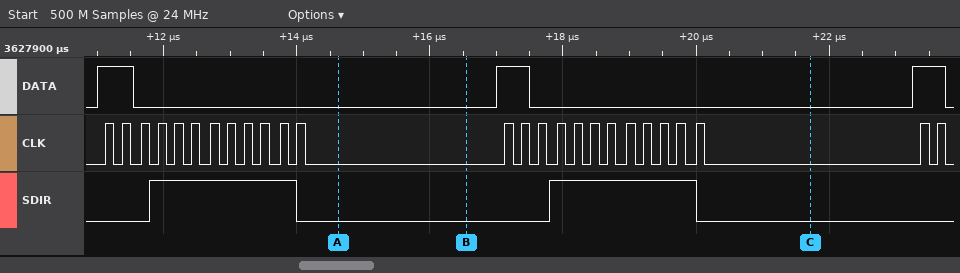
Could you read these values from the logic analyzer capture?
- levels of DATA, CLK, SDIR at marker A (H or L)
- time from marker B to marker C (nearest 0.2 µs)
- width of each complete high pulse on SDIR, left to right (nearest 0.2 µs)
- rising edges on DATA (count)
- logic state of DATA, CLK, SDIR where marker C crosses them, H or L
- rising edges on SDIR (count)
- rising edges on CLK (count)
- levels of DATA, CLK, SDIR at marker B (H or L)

DATA=L, CLK=L, SDIR=L
5.2 µs
2.2 µs, 2.2 µs
3
DATA=L, CLK=L, SDIR=L
2
26
DATA=L, CLK=L, SDIR=L
